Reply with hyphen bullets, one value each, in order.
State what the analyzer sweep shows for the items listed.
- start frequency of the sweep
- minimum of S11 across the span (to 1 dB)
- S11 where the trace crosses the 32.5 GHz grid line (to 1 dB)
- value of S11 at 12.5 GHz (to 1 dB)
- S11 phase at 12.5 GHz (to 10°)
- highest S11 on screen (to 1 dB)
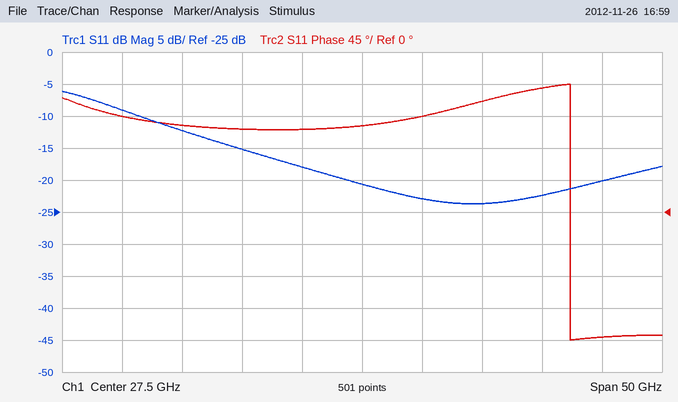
- 2.5 GHz
- -24 dB
- -23 dB
- -12 dB
- 120°
- -6 dB
